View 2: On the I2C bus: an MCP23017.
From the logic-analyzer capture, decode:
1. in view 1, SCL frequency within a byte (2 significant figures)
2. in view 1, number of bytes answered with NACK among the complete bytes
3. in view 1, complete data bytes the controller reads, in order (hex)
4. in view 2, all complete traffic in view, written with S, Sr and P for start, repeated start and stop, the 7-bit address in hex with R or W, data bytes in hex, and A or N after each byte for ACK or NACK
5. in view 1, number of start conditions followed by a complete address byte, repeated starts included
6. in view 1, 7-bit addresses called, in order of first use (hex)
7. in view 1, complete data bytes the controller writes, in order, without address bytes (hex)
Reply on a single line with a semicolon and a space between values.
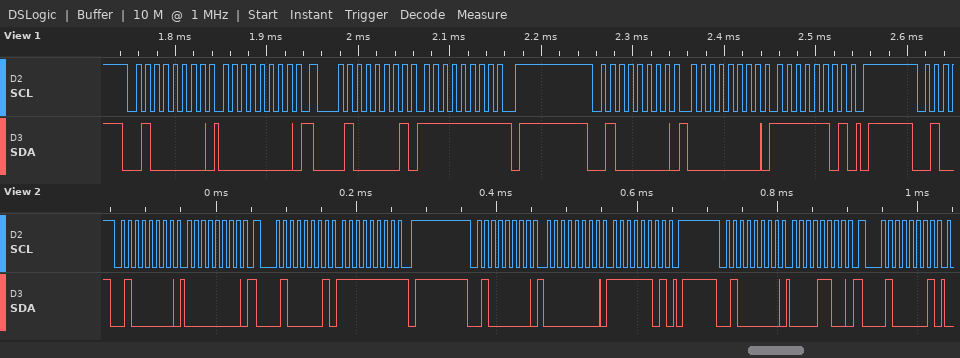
100 kHz; 1; FF; S 20W A 00 A Sr 20R A FF N P S 20W A 00 A FD A P S 20W A 0C A Sr 20R A; 3; 0x20; 00 00 FD
